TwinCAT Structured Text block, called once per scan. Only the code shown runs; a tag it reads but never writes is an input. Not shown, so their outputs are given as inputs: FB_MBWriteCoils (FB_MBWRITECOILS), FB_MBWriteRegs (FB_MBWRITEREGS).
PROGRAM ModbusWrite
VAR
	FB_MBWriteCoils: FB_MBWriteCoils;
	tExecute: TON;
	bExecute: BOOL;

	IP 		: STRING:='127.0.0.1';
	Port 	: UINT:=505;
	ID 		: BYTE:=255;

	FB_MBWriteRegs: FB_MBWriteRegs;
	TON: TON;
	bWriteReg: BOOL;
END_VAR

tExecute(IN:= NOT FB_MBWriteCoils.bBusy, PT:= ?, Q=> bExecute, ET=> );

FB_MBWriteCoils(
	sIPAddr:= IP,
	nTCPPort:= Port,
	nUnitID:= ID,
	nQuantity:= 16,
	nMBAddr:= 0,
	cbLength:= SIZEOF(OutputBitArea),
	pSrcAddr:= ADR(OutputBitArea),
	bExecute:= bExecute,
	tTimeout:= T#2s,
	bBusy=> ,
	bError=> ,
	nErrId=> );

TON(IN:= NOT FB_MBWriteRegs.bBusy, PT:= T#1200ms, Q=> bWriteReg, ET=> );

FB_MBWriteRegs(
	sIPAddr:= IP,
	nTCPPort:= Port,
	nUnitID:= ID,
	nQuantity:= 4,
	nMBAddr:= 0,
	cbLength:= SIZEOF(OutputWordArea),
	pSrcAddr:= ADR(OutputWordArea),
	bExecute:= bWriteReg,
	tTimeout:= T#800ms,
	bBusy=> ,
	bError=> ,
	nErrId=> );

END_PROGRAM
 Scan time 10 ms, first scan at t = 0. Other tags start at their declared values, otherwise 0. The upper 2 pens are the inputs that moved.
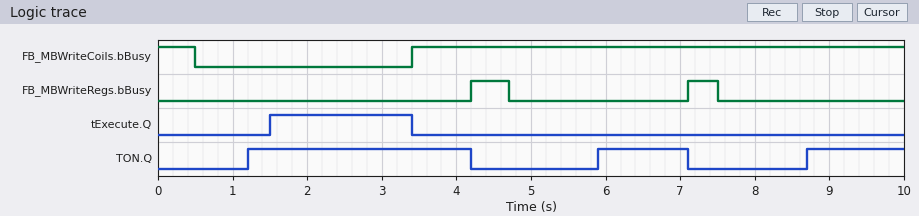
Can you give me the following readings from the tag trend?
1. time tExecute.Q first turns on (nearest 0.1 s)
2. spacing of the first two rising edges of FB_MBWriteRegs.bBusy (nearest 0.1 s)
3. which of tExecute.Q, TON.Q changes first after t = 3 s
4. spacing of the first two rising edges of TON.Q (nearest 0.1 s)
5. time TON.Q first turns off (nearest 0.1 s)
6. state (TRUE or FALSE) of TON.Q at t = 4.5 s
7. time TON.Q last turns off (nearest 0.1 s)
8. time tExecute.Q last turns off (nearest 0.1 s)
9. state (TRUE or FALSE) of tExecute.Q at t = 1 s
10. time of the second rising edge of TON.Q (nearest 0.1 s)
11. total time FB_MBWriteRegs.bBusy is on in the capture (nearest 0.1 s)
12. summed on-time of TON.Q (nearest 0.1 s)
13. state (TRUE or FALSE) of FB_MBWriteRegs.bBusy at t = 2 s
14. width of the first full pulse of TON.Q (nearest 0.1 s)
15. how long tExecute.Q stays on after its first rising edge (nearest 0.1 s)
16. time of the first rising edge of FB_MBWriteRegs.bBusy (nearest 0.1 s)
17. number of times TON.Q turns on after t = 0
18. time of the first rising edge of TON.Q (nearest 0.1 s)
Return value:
1.5 s
2.9 s
tExecute.Q
4.7 s
4.2 s
FALSE
7.1 s
3.4 s
FALSE
5.9 s
0.9 s
5.5 s
FALSE
3.0 s
1.9 s
4.2 s
3
1.2 s
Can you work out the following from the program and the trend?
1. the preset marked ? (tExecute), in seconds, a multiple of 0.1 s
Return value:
1.0 s
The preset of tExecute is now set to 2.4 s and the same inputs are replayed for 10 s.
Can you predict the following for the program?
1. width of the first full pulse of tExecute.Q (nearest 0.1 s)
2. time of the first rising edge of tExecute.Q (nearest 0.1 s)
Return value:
0.5 s
2.9 s
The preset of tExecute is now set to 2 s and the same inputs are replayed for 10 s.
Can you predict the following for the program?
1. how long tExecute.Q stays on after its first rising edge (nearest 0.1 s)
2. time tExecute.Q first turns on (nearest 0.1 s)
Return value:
0.9 s
2.5 s
